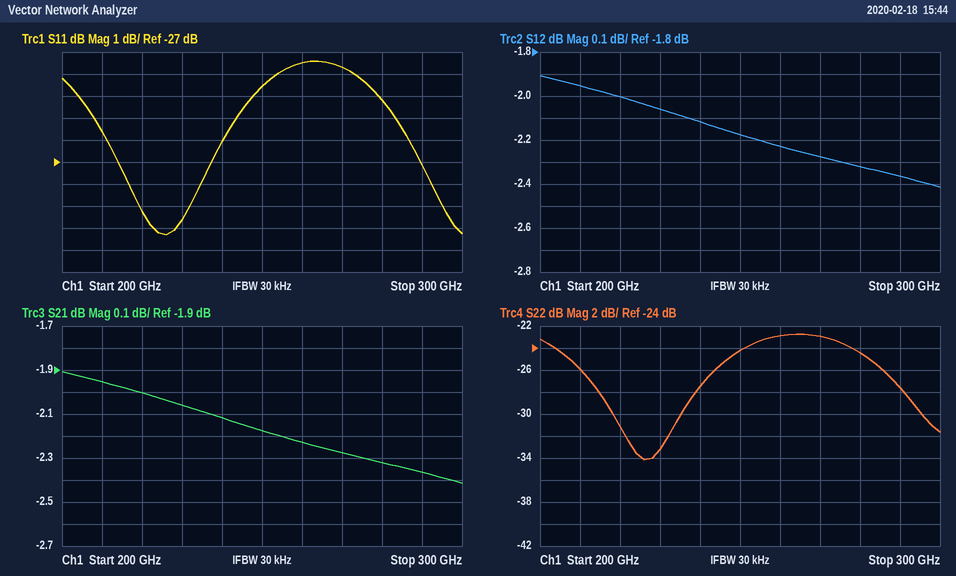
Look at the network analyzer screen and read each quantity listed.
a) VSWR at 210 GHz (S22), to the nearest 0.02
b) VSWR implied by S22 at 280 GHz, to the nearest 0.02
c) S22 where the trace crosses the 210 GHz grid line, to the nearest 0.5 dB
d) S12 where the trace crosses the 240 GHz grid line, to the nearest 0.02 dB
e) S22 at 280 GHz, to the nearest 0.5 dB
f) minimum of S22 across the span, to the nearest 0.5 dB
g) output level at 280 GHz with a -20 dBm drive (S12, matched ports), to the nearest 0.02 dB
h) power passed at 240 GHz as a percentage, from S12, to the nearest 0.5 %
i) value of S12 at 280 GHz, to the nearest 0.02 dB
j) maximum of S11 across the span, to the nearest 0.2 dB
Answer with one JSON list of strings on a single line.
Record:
["1.10", "1.12", "-26.0 dB", "-2.12 dB", "-24.5 dB", "-34.0 dB", "-22.32 dBm", "61.5 %", "-2.32 dB", "-22.4 dB"]
